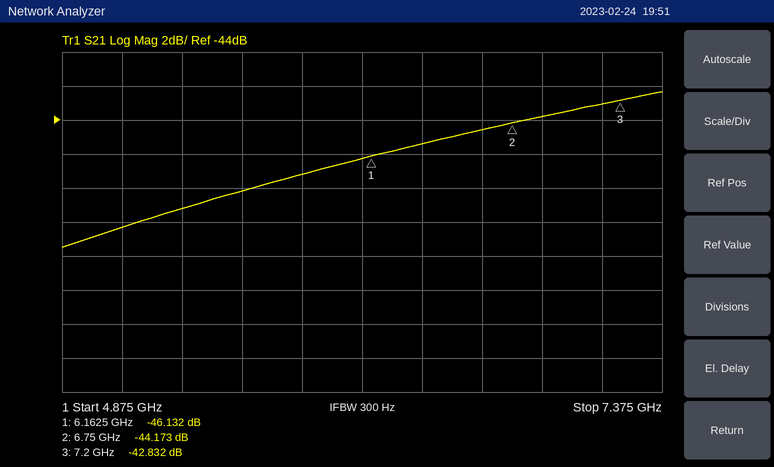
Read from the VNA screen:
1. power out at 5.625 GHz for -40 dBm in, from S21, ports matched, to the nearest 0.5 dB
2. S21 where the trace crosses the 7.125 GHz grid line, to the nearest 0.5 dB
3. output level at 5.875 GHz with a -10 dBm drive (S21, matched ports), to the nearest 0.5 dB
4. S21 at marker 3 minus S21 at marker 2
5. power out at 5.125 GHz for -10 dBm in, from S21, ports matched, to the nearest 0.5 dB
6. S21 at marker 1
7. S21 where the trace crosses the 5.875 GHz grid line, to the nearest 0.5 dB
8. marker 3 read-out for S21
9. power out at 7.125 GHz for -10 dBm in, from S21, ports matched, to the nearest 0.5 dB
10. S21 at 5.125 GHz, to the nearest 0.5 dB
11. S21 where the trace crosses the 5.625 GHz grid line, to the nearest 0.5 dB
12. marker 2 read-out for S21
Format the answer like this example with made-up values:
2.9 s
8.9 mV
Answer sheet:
-88.0 dBm
-43.0 dB
-57.0 dBm
1.341 dB
-60.5 dBm
-46.132 dB
-47.0 dB
-42.832 dB
-53.0 dBm
-50.5 dB
-48.0 dB
-44.173 dB
